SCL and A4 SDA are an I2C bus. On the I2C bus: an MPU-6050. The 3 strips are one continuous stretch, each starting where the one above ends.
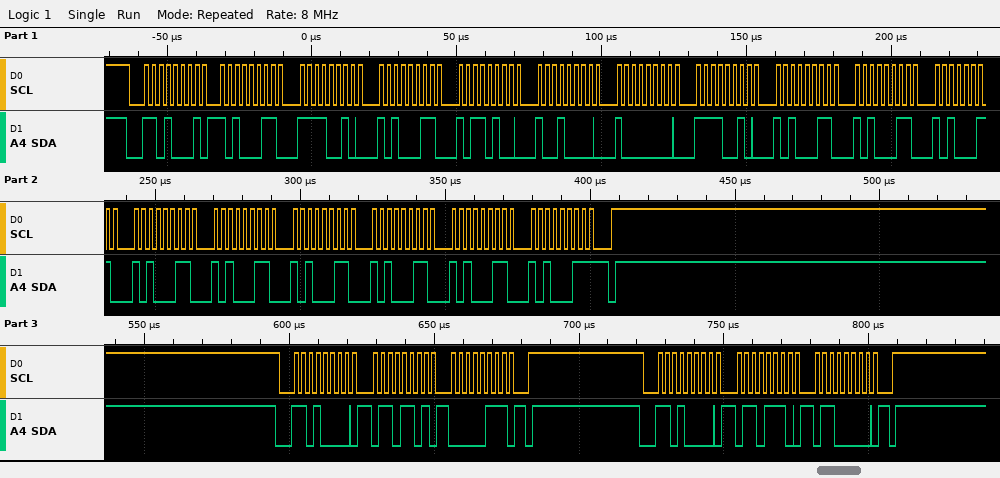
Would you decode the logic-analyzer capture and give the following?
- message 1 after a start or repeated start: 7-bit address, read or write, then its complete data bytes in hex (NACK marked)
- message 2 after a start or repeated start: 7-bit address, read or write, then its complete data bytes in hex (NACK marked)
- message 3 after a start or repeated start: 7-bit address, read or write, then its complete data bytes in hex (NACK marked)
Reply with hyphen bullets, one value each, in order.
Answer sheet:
- 0x68 read: A3 F2 A3 B4 90 80 F2 A3 A3 A3 A3 A3 A3 A3 A3 A3 NACK
- 0x68 write: 6D 07
- 0x68 write: 6E 60
